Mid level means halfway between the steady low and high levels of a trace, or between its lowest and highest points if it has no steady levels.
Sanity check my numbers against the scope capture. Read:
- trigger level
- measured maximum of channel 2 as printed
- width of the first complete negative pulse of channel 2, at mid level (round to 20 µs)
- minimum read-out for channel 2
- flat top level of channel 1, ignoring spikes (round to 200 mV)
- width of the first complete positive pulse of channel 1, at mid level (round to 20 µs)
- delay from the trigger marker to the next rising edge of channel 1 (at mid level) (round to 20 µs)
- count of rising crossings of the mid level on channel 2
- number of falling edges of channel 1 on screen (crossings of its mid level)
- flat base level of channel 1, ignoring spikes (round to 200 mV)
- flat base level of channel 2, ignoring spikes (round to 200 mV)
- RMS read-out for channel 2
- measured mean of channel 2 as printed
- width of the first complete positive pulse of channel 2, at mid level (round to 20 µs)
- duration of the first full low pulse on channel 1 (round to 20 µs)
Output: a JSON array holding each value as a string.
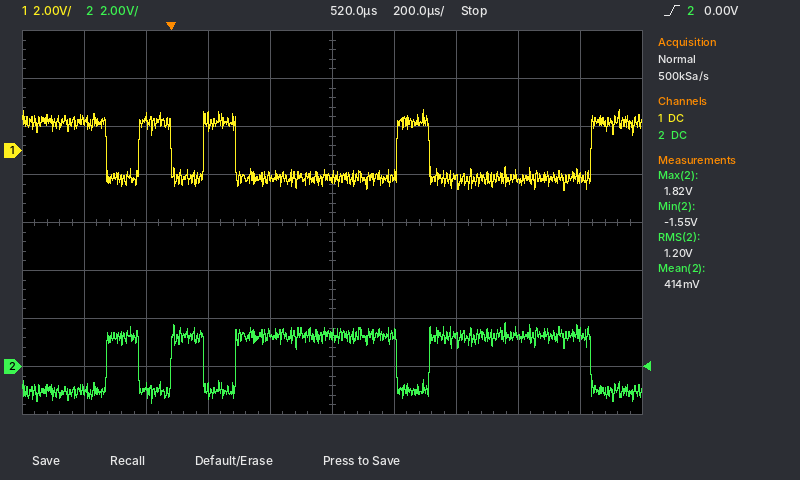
["0.00 V", "1.82 V", "100 µs", "-1.55 V", "1.2 V", "100 µs", "100 µs", "4", "4", "-1.2 V", "-1.0 V", "1.20 V", "414 mV", "100 µs", "100 µs"]
